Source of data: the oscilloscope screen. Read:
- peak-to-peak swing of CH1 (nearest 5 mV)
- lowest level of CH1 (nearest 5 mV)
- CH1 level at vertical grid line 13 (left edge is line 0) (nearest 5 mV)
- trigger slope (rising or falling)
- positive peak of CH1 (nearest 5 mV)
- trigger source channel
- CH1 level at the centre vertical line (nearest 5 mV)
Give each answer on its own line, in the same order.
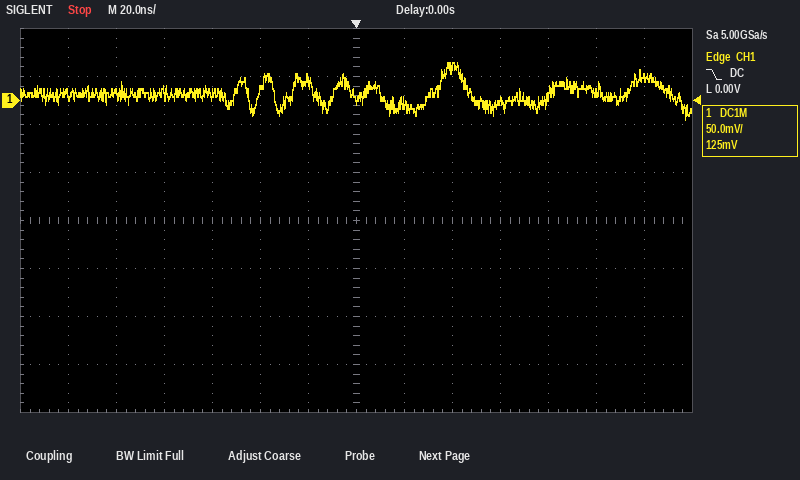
60 mV
-20 mV
25 mV
falling
40 mV
CH1
0 mV
